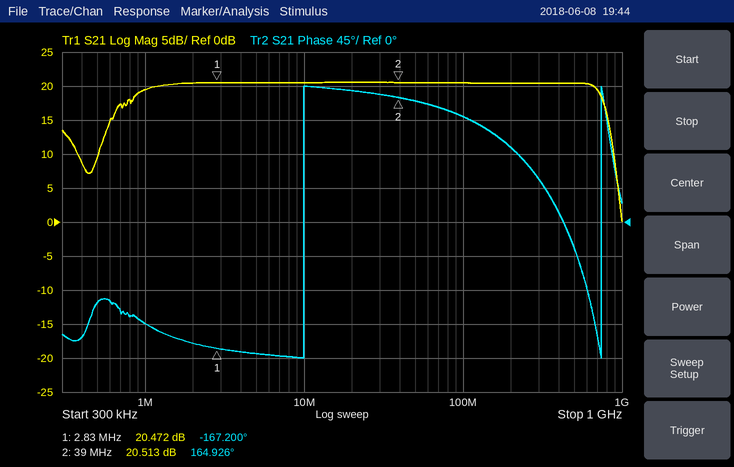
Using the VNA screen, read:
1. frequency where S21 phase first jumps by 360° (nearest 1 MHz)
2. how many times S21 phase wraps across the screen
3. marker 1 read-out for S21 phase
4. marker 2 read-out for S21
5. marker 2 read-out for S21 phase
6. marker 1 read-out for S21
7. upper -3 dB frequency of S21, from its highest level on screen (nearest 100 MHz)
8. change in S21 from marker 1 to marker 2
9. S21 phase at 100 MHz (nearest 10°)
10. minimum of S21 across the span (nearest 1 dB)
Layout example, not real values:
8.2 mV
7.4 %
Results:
10 MHz
2
-167.200°
20.513 dB
164.926°
20.472 dB
800 MHz
0.041 dB
140°
0 dB
